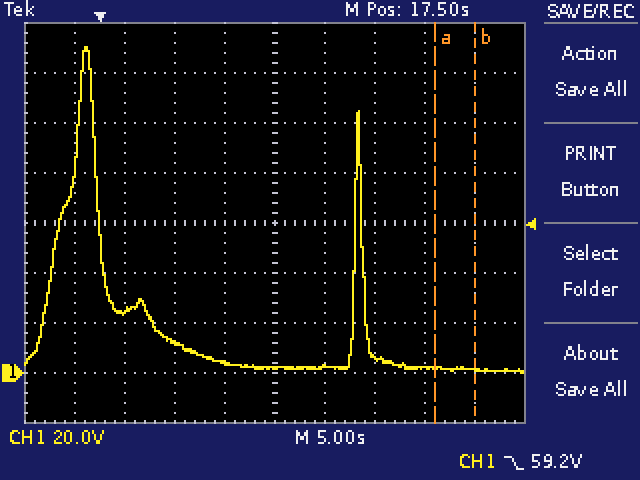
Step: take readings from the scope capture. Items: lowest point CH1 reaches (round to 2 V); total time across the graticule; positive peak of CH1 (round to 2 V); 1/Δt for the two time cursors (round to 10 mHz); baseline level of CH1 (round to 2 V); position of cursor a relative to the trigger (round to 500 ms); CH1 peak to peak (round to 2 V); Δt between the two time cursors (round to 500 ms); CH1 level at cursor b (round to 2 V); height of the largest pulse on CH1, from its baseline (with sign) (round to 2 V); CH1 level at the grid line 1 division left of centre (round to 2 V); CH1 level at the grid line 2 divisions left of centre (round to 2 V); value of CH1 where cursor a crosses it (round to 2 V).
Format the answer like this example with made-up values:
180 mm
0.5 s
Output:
0 V
50 s
130 V
250 mHz
2 V
+33.5 s
130 V
4.0 s
2 V
+128 V
4 V
12 V
2 V
